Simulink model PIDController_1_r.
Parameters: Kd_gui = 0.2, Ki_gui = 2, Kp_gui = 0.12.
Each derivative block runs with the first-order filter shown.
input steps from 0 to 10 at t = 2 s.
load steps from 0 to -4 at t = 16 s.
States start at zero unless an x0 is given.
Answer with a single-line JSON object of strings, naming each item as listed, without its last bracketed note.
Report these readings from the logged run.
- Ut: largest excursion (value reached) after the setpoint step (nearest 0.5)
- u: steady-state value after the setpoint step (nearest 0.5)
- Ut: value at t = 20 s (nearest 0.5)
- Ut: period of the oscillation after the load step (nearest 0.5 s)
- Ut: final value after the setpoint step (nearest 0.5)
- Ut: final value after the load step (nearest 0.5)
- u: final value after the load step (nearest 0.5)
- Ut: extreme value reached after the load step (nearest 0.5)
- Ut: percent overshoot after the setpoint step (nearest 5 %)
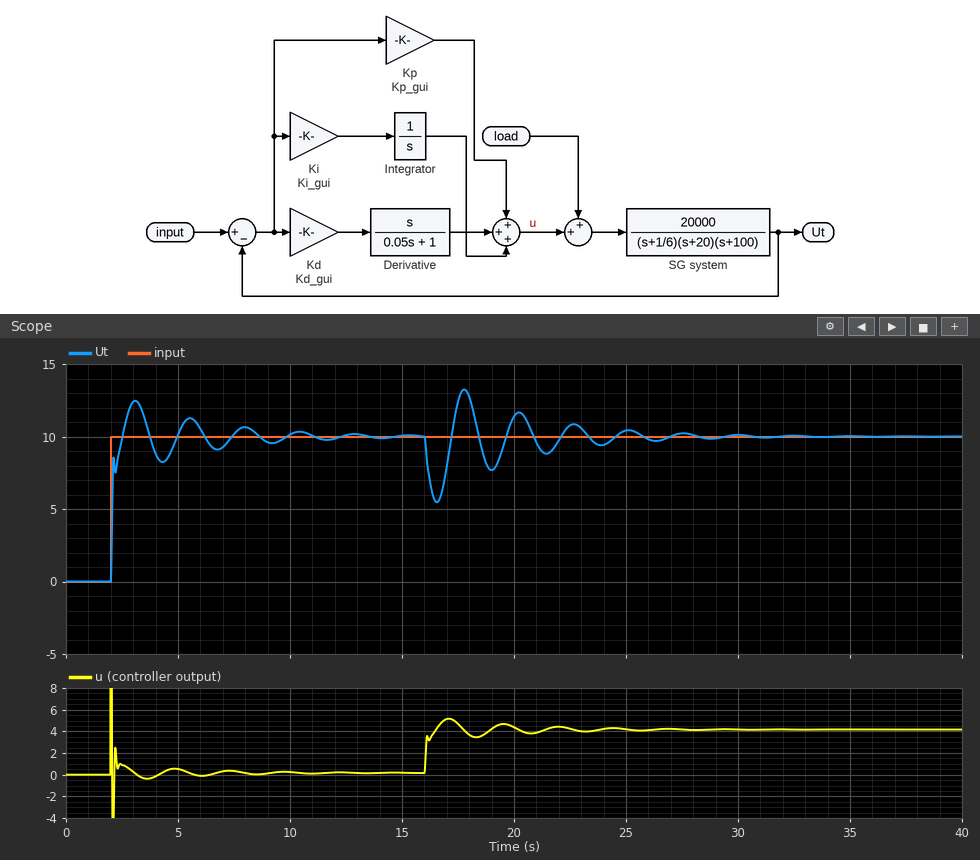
{"Ut: largest excursion (value reached) after the setpoint step": "12.5", "u: steady-state value after the setpoint step": "0.0", "Ut: value at t = 20 s": "11.5", "Ut: period of the oscillation after the load step": "2.5 s", "Ut: final value after the setpoint step": "10.0", "Ut: final value after the load step": "10.0", "u: final value after the load step": "4.0", "Ut: extreme value reached after the load step": "5.5", "Ut: percent overshoot after the setpoint step": "25 %"}
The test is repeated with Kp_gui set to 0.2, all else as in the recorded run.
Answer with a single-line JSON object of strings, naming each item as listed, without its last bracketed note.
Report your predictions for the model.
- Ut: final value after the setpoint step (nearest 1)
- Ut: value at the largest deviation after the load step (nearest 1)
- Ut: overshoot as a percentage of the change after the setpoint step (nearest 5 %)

{"Ut: final value after the setpoint step": "10", "Ut: value at the largest deviation after the load step": "6", "Ut: overshoot as a percentage of the change after the setpoint step": "20 %"}
